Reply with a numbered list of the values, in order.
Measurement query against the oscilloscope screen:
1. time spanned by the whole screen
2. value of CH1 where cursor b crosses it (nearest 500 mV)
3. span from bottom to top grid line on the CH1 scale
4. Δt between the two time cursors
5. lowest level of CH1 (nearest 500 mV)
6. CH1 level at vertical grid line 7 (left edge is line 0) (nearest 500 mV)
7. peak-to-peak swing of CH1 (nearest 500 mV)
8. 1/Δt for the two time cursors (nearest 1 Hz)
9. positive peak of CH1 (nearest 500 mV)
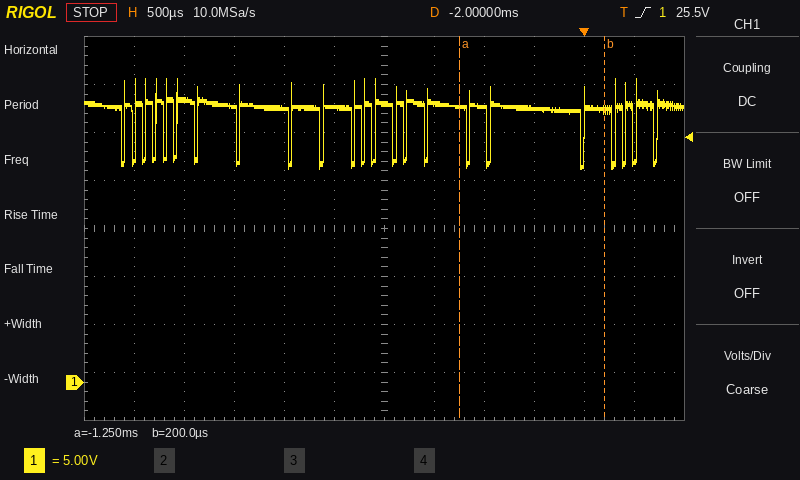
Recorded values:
1. 6 ms
2. 28.5 V
3. 40 V
4. 1.45 ms
5. 22.0 V
6. 29.0 V
7. 9.5 V
8. 690 Hz
9. 31.5 V
